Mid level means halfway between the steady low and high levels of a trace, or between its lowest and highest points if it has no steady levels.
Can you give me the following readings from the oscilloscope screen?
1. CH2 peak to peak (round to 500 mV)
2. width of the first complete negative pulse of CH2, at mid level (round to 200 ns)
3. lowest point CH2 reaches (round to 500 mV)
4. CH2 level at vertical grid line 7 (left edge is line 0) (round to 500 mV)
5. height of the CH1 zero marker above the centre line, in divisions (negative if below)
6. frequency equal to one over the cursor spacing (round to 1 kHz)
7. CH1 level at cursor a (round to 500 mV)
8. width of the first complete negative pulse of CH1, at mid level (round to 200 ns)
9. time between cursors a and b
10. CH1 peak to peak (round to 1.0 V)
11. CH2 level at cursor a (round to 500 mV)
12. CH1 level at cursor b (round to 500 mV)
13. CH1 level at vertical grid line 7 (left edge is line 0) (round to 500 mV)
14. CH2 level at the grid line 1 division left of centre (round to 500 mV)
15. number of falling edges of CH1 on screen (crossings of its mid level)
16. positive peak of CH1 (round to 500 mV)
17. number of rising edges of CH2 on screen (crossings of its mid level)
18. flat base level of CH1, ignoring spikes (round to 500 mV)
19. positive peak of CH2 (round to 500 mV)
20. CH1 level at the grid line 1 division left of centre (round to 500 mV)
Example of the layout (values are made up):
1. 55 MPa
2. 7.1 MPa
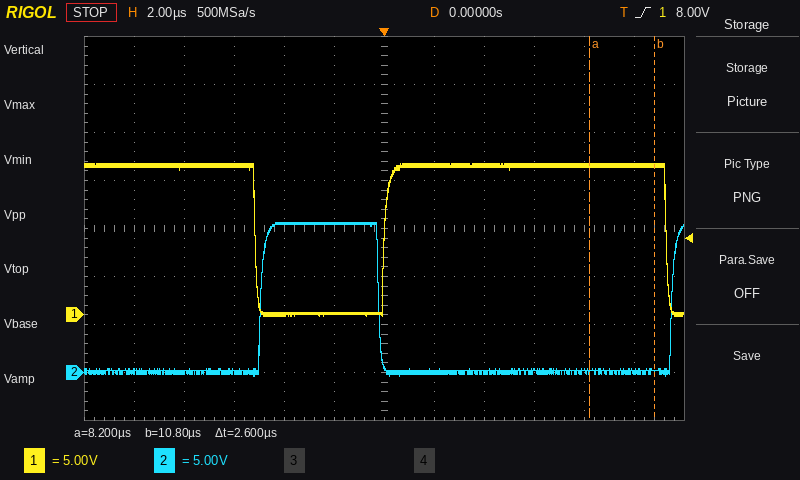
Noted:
1. 16.0 V
2. 11.8 µs
3. -500 mV
4. 0.0 V
5. -1.8 div
6. 385 kHz
7. 15.5 V
8. 5.2 µs
9. 2.6 µs
10. 16.0 V
11. 0.0 V
12. 15.5 V
13. 15.5 V
14. 15.5 V
15. 2
16. 16.0 V
17. 2
18. 0.0 V
19. 15.5 V
20. 0.0 V
